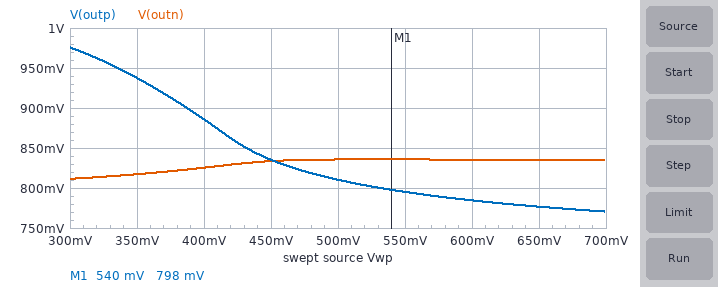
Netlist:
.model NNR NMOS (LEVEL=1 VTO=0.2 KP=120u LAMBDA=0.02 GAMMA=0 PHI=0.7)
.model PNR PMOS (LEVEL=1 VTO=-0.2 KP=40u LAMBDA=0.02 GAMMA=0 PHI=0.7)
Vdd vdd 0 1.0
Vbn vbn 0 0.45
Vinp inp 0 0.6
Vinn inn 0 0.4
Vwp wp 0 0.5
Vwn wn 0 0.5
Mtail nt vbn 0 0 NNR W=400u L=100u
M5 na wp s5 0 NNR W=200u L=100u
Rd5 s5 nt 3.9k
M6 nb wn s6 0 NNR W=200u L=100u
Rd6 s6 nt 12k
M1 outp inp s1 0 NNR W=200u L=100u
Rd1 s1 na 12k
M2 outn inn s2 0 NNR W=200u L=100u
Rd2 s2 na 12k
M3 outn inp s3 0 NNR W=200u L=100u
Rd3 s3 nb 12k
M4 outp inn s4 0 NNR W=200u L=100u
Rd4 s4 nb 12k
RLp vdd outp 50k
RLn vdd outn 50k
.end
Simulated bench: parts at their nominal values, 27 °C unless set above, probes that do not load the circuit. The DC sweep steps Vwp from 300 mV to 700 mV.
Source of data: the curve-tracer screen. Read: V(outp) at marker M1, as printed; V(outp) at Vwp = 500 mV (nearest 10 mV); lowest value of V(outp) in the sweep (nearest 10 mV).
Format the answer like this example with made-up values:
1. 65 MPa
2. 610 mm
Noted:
1. 798 mV
2. 810 mV
3. 770 mV
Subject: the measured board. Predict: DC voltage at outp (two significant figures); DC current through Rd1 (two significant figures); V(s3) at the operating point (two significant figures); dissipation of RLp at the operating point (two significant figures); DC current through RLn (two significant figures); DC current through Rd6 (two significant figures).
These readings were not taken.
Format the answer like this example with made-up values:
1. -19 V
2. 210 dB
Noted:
1. 810 mV
2. 3.8 µA
3. 240 mV
4. 720 nW
5. 3.3 µA
6. 3.2 µA
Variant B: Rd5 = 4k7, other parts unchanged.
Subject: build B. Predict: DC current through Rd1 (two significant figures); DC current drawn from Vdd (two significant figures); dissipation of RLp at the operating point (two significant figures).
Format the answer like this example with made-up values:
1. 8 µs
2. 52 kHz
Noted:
1. 3.7 µA
2. 7.0 µA
3. 700 nW
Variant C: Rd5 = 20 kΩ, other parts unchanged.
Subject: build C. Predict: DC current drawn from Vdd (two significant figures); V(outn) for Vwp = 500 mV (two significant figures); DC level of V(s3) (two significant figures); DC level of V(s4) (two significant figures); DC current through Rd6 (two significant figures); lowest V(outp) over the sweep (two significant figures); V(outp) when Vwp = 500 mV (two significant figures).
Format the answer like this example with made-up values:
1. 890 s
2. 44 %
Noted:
1. 6.3 µA
2. 830 mV
3. 230 mV
4. 190 mV
5. 3.4 µA
6. 820 mV
7. 850 mV
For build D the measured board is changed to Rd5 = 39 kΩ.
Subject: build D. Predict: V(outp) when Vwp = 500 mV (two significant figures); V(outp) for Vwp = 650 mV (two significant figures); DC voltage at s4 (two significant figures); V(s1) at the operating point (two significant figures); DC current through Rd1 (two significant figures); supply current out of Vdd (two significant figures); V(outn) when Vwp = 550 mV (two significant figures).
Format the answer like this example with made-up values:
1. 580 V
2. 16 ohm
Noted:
1. 880 mV
2. 860 mV
3. 190 mV
4. 260 mV
5. 2.3 µA
6. 5.8 µA
7. 830 mV
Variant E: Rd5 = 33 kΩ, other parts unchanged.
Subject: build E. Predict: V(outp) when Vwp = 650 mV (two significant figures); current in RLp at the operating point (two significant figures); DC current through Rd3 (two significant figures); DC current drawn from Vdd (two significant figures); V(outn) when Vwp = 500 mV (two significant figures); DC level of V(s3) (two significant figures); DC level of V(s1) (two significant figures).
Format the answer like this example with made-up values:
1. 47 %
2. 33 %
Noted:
1. 850 mV
2. 2.5 µA
3. 3.5 µA
4. 6.0 µA
5. 830 mV
6. 230 mV
7. 260 mV
